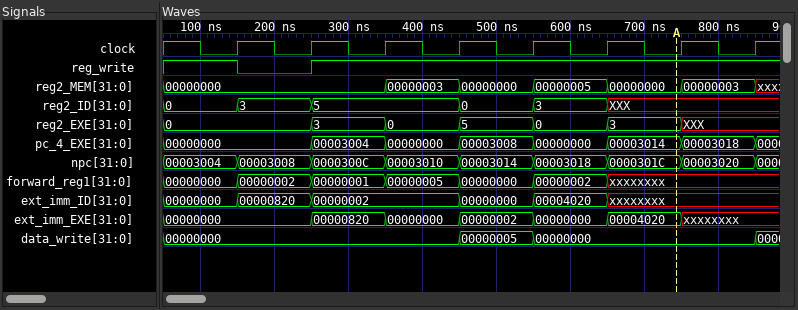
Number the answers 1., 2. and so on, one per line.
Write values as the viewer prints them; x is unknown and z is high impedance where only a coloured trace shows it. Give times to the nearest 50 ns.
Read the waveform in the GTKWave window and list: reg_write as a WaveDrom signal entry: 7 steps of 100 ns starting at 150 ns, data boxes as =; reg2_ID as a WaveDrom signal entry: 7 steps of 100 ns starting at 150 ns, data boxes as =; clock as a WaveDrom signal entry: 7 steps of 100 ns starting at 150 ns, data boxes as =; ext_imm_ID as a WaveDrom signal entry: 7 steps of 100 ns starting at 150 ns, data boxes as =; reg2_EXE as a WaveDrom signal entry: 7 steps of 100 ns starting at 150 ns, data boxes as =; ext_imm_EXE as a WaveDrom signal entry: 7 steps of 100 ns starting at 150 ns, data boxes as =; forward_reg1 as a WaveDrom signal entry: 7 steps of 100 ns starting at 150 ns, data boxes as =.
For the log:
1. {name: 'reg_write', wave: '01.....'}
2. {name: 'reg2_ID', wave: '==.==x.', data: '3 5 0 3'}
3. {name: 'clock', wave: 'p......'}
4. {name: 'ext_imm_ID', wave: '==.==x.', data: '00000820 00000002 00000000 00004020'}
5. {name: 'reg2_EXE', wave: '======x', data: '0 3 0 5 0 3'}
6. {name: 'ext_imm_EXE', wave: '======x', data: '00000000 00000820 00000000 00000002 00000000 00004020'}
7. {name: 'forward_reg1', wave: '=====x.', data: '00000002 00000001 00000005 00000000 00000002'}
